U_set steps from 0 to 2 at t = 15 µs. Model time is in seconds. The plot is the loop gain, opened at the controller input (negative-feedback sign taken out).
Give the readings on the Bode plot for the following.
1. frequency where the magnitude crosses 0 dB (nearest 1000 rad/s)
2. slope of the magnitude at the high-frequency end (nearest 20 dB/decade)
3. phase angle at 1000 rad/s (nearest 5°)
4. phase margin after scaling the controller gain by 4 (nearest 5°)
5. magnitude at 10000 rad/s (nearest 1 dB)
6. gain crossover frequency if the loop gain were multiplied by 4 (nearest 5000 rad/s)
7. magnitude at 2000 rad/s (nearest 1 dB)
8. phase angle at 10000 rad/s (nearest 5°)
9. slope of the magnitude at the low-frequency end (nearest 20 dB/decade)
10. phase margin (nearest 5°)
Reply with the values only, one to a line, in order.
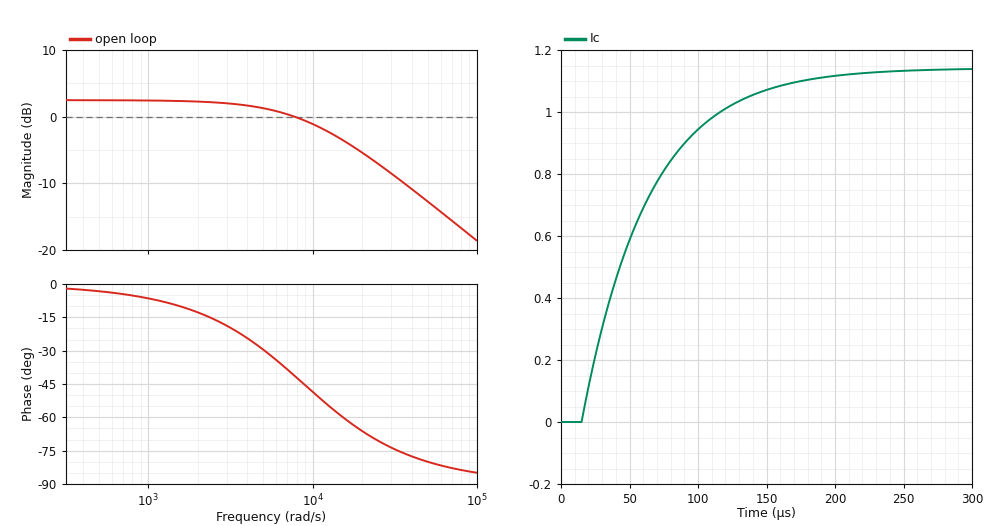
8000 rad/s
-20 dB/decade
-5°
100°
-1 dB
45000 rad/s
2 dB
-50°
0 dB/decade
140°
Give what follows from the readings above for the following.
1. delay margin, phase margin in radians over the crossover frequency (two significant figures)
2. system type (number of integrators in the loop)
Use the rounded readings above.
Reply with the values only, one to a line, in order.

0.00031 s
0
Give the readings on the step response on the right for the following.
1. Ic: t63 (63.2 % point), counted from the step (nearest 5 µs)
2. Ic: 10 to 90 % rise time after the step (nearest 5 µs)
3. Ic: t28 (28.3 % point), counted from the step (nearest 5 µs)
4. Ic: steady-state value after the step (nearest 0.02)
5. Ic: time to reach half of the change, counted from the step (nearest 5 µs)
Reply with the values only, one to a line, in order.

50 µs
105 µs
15 µs
1.14
35 µs
